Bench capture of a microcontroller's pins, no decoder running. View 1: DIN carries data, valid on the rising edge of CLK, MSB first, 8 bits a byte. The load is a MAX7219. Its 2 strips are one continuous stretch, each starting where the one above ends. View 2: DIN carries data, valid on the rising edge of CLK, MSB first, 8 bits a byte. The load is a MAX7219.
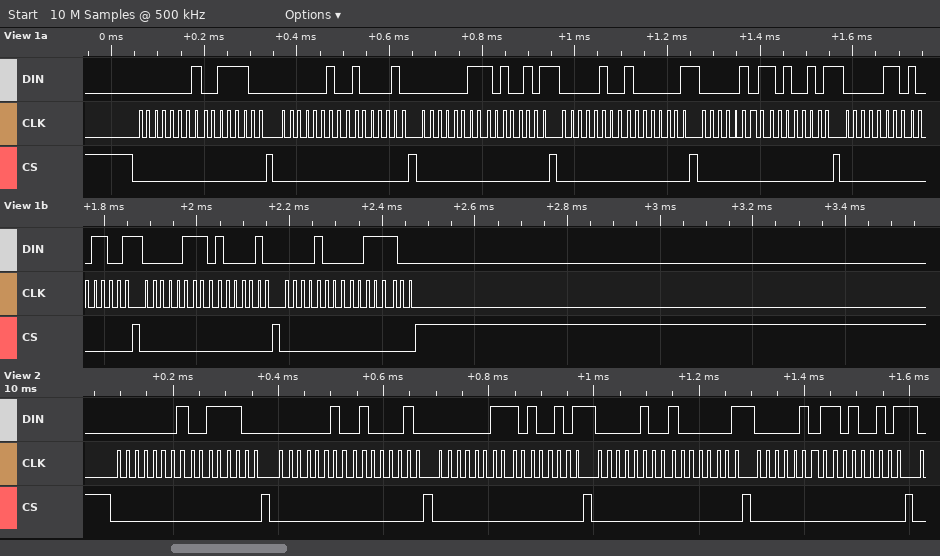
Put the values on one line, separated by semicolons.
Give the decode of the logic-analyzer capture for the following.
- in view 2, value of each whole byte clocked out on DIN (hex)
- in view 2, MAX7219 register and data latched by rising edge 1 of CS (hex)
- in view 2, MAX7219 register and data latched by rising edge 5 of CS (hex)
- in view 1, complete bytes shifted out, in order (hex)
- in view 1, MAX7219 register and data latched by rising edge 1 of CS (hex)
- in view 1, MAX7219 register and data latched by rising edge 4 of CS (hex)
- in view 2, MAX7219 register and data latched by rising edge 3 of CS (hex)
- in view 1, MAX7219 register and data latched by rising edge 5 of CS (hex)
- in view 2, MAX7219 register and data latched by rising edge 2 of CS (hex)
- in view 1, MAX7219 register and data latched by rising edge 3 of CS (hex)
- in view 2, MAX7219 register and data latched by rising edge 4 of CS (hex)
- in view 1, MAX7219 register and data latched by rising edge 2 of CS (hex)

01 3C 02 42 03 A5 04 81 05 A5; register 0x1, data 0x3C; register 0x5, data 0xA5; 0x01 0x3C 0x02 0x42 0x03 0xA5 0x04 0x81 0x05 0xA5 0x06 0x99 0x07 0x42 0x08 0x3C; register 0x1, data 0x3C; register 0x4, data 0x81; register 0x3, data 0xA5; register 0x5, data 0xA5; register 0x2, data 0x42; register 0x3, data 0xA5; register 0x4, data 0x81; register 0x2, data 0x42
